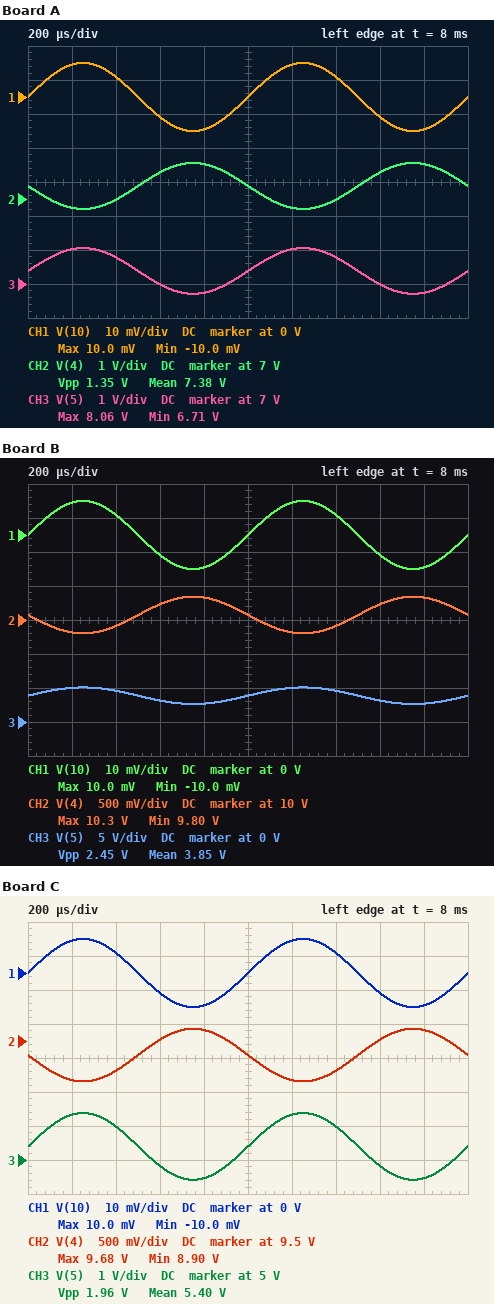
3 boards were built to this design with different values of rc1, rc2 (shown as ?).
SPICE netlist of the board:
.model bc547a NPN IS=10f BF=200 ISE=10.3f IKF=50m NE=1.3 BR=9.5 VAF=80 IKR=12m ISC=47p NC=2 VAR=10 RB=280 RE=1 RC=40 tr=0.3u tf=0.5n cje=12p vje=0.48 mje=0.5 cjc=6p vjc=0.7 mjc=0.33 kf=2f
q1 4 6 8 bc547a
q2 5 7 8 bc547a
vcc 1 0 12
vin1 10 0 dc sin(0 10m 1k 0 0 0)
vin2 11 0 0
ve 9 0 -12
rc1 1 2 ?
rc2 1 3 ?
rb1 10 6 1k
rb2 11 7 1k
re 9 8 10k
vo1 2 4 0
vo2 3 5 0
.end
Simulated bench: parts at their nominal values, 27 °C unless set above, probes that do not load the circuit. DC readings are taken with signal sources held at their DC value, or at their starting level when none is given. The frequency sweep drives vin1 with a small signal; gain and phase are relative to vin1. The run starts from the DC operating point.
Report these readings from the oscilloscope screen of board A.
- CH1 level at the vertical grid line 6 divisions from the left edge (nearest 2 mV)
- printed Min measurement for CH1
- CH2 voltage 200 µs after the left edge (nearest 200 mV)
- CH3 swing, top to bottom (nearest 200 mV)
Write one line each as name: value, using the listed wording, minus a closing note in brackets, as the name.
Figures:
CH1 level at the vertical grid line 6 divisions from the left edge: 10 mV
printed Min measurement for CH1: -10.0 mV
CH2 voltage 200 µs after the left edge: 6.8 V
CH3 swing, top to bottom: 1.4 V
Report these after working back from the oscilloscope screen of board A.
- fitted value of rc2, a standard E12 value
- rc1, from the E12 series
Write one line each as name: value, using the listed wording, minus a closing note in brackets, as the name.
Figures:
fitted value of rc2, a standard E12 value: 8.2 kΩ
rc1, from the E12 series: 8.2 kΩ
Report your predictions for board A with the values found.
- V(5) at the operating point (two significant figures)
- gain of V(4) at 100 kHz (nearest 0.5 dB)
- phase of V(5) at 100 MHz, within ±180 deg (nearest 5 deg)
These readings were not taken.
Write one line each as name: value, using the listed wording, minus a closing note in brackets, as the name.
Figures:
V(5) at the operating point: 7.4 V
gain of V(4) at 100 kHz: 36.0 dB
phase of V(5) at 100 MHz, within ±180 deg: -10 deg
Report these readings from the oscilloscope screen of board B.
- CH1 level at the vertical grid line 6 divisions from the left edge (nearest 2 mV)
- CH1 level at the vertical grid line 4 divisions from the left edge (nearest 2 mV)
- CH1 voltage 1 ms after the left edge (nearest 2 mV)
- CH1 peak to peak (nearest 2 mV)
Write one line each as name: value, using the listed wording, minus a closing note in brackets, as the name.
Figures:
CH1 level at the vertical grid line 6 divisions from the left edge: 10 mV
CH1 level at the vertical grid line 4 divisions from the left edge: -10 mV
CH1 voltage 1 ms after the left edge: 0 V
CH1 peak to peak: 20 mV
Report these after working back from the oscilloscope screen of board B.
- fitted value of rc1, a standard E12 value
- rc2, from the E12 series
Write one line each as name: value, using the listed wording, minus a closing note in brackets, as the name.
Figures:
fitted value of rc1, a standard E12 value: 3.3 kΩ
rc2, from the E12 series: 15 kΩ
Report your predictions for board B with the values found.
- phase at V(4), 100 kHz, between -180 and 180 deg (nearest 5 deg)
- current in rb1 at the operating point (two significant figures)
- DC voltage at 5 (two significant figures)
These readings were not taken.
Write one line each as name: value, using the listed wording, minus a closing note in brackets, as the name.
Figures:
phase at V(4), 100 kHz, between -180 and 180 deg: 160 deg
current in rb1 at the operating point: 4.7 µA
DC voltage at 5: 3.9 V
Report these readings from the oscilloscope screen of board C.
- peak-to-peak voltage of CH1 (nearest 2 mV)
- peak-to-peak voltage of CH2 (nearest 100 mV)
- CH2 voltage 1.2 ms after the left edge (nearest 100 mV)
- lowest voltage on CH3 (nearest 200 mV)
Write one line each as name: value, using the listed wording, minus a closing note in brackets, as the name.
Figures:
peak-to-peak voltage of CH1: 20 mV
peak-to-peak voltage of CH2: 800 mV
CH2 voltage 1.2 ms after the left edge: 8.9 V
lowest voltage on CH3: 4.4 V
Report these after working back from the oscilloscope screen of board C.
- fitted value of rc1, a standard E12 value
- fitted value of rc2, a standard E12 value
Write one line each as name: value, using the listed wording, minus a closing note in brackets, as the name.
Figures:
fitted value of rc1, a standard E12 value: 4.7 kΩ
fitted value of rc2, a standard E12 value: 12 kΩ
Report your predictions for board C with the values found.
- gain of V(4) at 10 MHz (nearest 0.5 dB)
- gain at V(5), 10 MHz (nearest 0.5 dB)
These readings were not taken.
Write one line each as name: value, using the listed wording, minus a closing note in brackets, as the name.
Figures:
gain of V(4) at 10 MHz: 6.0 dB
gain at V(5), 10 MHz: 6.0 dB
